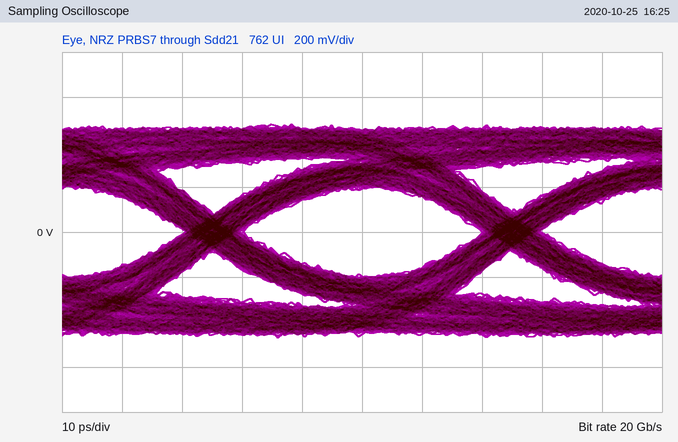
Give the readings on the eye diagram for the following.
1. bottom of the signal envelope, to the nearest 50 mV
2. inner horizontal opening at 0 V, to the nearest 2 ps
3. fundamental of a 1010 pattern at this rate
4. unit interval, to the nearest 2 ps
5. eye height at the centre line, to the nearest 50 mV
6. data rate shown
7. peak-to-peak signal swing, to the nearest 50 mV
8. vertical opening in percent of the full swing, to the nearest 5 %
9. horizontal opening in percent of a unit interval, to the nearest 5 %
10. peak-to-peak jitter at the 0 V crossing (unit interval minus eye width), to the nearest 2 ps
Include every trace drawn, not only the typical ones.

-450 mV
40 ps
10 GHz
50 ps
400 mV
20 Gb/s
950 mV
40 %
80 %
10 ps
